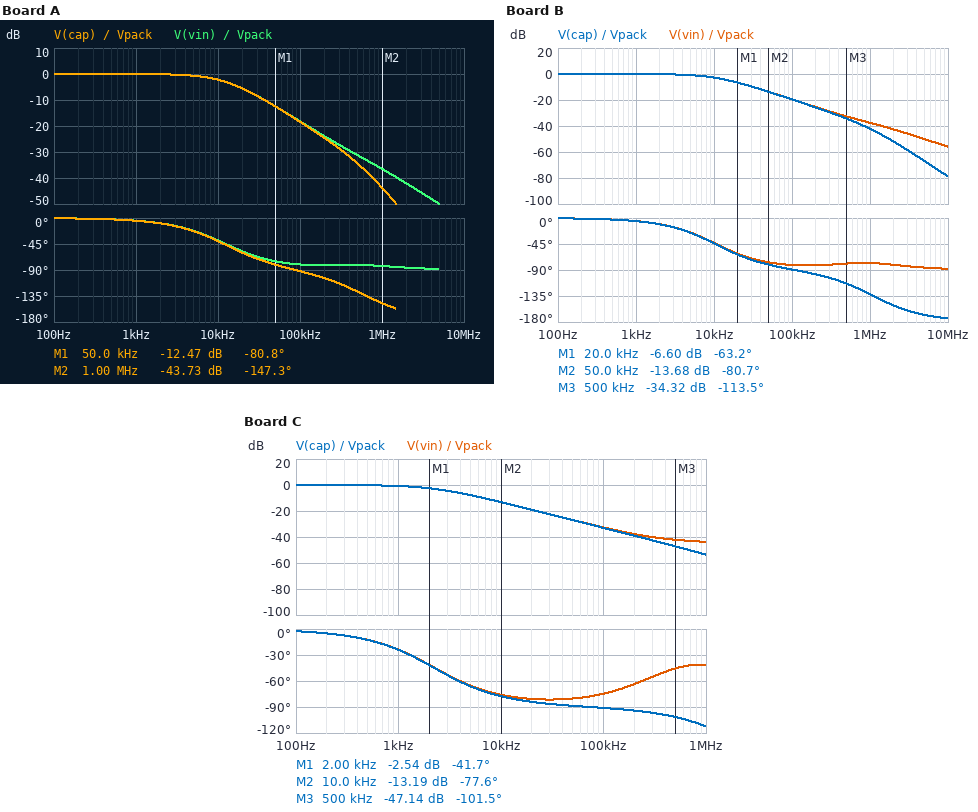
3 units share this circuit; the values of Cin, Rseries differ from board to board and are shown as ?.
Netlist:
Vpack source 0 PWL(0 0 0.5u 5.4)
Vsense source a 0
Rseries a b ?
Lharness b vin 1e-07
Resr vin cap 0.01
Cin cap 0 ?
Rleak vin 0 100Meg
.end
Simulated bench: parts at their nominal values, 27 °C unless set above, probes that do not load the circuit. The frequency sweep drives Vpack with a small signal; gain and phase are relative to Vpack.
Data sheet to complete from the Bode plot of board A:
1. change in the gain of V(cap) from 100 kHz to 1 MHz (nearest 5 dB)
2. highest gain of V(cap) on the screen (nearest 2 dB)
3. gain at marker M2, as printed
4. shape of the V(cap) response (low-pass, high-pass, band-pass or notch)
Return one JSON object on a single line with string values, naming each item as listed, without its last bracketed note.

{"change in the gain of V(cap) from 100 kHz to 1 MHz": "-25 dB", "highest gain of V(cap) on the screen": "0 dB", "gain at marker M2, as printed": "-43.73 dB", "shape of the V(cap) response": "low-pass"}
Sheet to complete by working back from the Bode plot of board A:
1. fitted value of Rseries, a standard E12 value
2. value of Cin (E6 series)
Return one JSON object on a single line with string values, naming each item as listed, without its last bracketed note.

{"fitted value of Rseries, a standard E12 value": "0.39 Ω", "value of Cin": "33 µF"}
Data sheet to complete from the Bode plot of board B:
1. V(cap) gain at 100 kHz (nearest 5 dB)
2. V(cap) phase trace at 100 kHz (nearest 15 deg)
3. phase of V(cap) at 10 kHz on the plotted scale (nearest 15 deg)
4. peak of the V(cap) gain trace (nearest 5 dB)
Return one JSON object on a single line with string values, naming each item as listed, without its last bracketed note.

{"V(cap) gain at 100 kHz": "-20 dB", "V(cap) phase trace at 100 kHz": "-90 deg", "phase of V(cap) at 10 kHz on the plotted scale": "-45 deg", "peak of the V(cap) gain trace": "0 dB"}
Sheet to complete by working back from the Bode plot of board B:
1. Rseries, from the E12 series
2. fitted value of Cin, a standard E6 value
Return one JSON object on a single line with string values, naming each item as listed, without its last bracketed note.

{"Rseries, from the E12 series": "0.68 Ω", "fitted value of Cin, a standard E6 value": "22 µF"}
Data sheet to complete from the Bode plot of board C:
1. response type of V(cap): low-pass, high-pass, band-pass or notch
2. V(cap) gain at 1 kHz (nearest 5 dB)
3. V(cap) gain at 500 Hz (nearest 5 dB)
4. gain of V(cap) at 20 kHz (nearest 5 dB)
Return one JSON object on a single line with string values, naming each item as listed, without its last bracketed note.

{"response type of V(cap): low-pass, high-pass, band-pass or notch": "low-pass", "V(cap) gain at 1 kHz": "0 dB", "V(cap) gain at 500 Hz": "0 dB", "gain of V(cap) at 20 kHz": "-20 dB"}
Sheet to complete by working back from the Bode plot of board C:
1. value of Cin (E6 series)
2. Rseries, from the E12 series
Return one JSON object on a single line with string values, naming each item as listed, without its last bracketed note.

{"value of Cin": "47 µF", "Rseries, from the E12 series": "1.5 Ω"}
